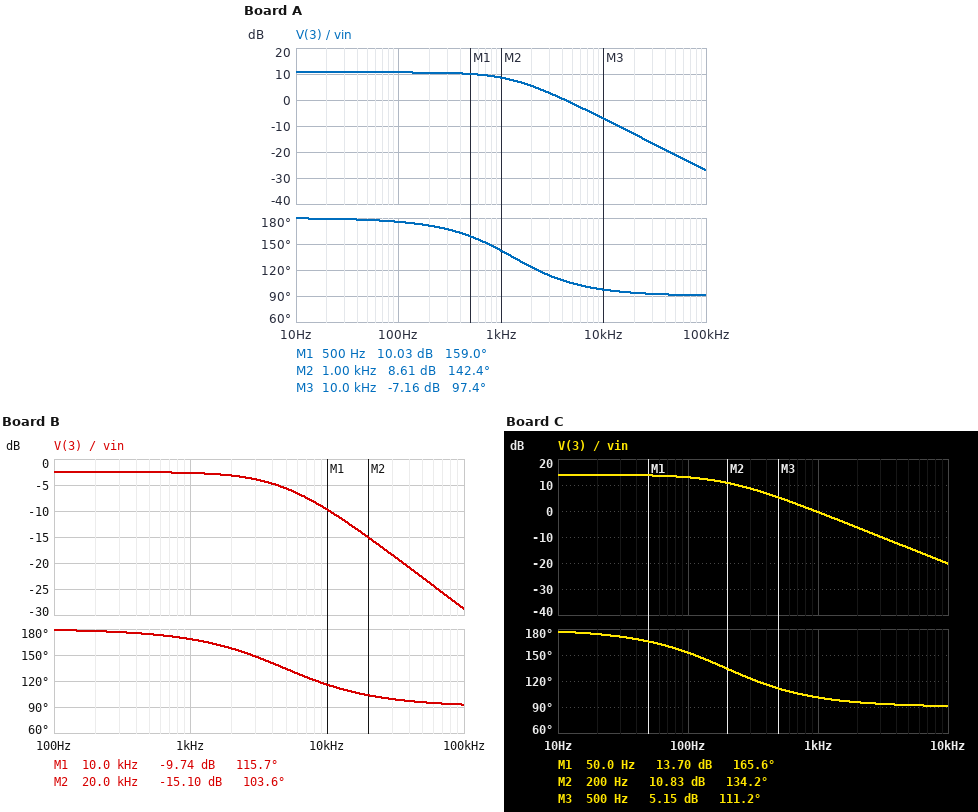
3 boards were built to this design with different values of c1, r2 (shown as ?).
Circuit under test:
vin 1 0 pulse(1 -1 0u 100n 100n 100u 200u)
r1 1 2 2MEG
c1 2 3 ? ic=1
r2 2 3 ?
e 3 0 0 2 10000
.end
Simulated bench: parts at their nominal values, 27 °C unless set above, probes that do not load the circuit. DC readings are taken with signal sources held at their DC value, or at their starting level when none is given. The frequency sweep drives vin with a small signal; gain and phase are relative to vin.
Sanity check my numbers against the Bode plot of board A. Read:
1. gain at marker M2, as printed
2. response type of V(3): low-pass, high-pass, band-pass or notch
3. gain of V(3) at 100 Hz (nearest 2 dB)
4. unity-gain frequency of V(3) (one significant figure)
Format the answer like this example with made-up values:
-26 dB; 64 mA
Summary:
8.61 dB; low-pass; 10 dB; 4 kHz
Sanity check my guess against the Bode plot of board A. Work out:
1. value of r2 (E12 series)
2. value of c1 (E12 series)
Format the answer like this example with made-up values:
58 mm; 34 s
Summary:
6.8 MΩ; 18 pF
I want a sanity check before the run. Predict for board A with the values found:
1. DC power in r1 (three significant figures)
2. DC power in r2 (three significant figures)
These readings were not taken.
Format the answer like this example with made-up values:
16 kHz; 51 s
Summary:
500 nW; 1.70 µW
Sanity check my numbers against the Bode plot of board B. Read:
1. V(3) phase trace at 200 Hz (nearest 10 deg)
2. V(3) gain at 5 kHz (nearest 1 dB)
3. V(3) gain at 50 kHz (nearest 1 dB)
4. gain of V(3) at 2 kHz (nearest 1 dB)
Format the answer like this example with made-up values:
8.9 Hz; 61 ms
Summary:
180 deg; -6 dB; -23 dB; -3 dB
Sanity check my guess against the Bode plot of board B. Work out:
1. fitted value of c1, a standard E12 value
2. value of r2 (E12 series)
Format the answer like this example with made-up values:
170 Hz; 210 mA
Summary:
22 pF; 1.5 MΩ
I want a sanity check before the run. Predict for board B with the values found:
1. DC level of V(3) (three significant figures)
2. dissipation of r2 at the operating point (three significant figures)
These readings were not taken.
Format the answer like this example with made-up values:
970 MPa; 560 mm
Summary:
-750 mV; 375 nW
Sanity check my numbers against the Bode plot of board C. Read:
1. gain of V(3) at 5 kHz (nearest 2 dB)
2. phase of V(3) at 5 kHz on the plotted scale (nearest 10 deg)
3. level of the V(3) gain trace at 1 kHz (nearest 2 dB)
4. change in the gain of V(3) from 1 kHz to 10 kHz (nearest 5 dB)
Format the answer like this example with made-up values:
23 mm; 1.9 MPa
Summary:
-14 dB; 90 deg; 0 dB; -20 dB
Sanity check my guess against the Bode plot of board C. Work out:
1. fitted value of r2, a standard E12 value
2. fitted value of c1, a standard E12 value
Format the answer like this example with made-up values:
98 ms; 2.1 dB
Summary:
10 MΩ; 82 pF
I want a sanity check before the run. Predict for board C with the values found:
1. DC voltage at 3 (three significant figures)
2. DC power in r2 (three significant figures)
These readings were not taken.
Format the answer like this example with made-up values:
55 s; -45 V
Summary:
-5.00 V; 2.50 µW
